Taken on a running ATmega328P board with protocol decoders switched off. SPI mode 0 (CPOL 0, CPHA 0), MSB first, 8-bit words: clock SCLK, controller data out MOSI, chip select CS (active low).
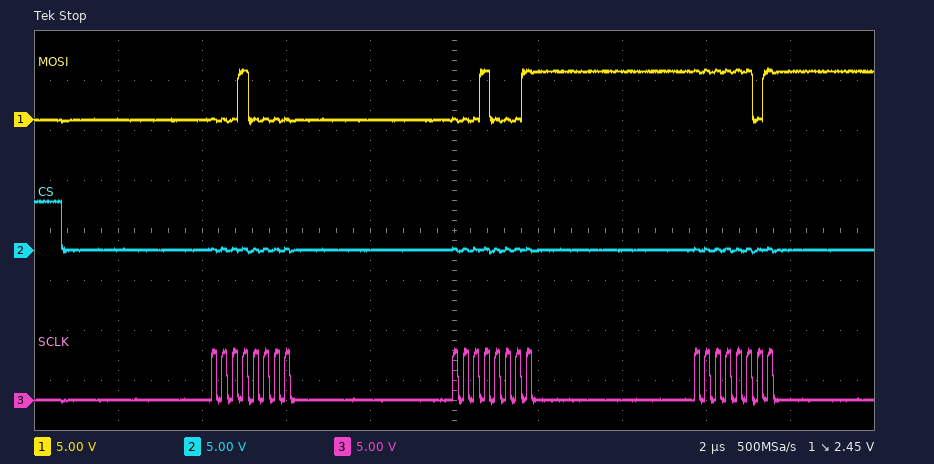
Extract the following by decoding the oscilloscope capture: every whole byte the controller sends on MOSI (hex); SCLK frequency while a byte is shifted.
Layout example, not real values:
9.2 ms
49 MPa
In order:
0x10 0x11 0xFD
4 MHz
